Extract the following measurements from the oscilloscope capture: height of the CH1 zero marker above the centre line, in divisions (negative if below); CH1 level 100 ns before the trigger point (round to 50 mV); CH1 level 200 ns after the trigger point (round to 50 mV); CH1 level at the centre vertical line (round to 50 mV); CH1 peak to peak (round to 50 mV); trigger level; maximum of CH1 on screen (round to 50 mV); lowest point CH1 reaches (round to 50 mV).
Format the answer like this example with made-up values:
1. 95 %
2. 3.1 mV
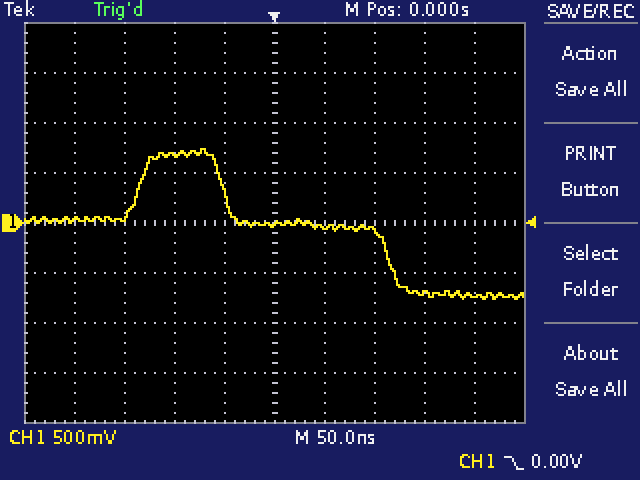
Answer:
1. 0.0 div
2. 700 mV
3. -750 mV
4. 0 mV
5. 1.50 V
6. 0.00 V
7. 750 mV
8. -750 mV
